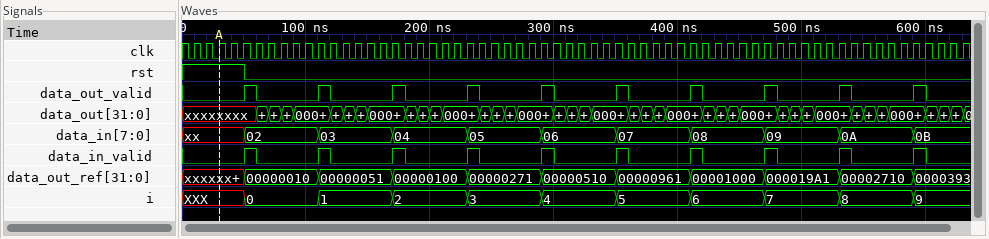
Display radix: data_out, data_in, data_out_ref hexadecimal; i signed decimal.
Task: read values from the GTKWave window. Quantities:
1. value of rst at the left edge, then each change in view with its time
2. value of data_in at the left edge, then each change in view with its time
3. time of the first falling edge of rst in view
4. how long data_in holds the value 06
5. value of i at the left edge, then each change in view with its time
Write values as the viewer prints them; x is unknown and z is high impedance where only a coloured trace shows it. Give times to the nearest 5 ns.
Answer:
1, 0 at 50 ns
xx, 02 at 50 ns, 03 at 110 ns, 04 at 170 ns, 05 at 230 ns, 06 at 290 ns, 07 at 350 ns, 08 at 410 ns, 09 at 470 ns, 0A at 530 ns, 0B at 590 ns
50 ns
60 ns
XXX, 0 at 50 ns, 1 at 110 ns, 2 at 170 ns, 3 at 230 ns, 4 at 290 ns, 5 at 350 ns, 6 at 410 ns, 7 at 470 ns, 8 at 530 ns, 9 at 590 ns
